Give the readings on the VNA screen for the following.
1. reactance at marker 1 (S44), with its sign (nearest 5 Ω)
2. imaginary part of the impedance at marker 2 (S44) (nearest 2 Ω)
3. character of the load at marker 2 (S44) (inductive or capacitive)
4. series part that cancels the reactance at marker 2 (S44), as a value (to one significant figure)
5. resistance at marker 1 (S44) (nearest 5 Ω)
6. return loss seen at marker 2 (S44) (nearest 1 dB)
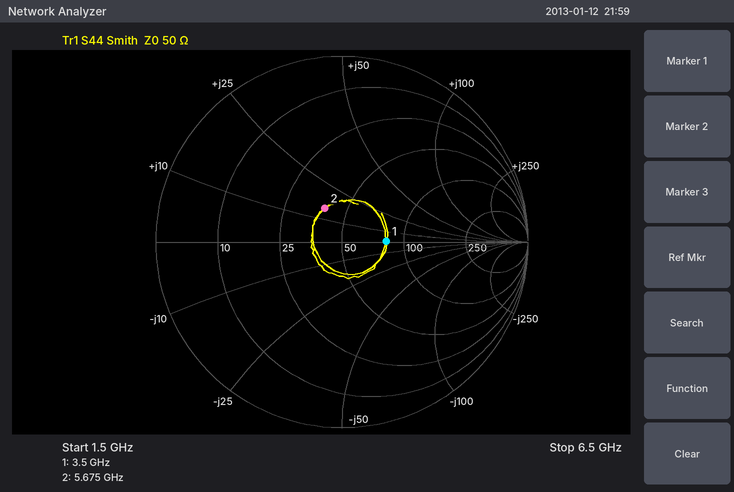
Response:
0 Ω
+14 Ω
inductive
2 pF
80 Ω
14 dB
